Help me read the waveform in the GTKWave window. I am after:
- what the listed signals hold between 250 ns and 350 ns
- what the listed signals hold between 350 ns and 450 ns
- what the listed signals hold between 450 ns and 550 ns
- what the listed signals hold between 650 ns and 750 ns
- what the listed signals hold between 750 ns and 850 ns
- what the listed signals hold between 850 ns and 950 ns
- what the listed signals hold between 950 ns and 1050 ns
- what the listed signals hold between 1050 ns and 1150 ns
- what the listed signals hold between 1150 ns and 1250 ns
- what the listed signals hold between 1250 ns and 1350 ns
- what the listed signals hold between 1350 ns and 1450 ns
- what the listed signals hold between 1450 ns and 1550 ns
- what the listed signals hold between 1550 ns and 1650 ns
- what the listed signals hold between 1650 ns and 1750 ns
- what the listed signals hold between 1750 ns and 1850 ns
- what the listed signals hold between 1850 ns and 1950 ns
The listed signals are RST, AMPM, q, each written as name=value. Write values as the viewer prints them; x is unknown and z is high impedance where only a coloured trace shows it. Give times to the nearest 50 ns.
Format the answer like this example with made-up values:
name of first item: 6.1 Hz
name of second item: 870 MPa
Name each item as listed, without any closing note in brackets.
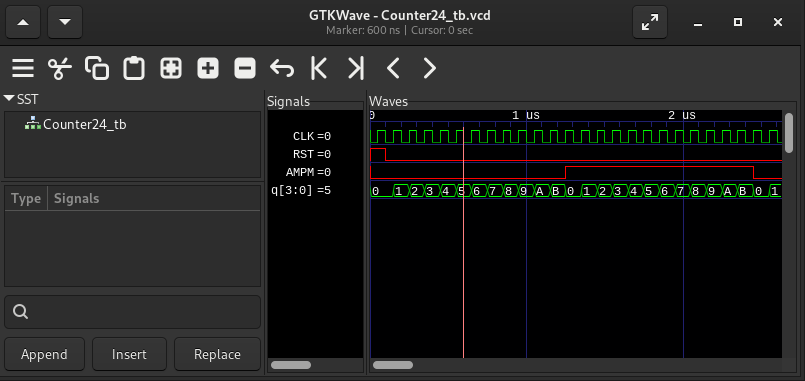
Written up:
what the listed signals hold between 250 ns and 350 ns: RST=0, AMPM=0, q=2
what the listed signals hold between 350 ns and 450 ns: RST=0, AMPM=0, q=3
what the listed signals hold between 450 ns and 550 ns: RST=0, AMPM=0, q=4
what the listed signals hold between 650 ns and 750 ns: RST=0, AMPM=0, q=6
what the listed signals hold between 750 ns and 850 ns: RST=0, AMPM=0, q=7
what the listed signals hold between 850 ns and 950 ns: RST=0, AMPM=0, q=8
what the listed signals hold between 950 ns and 1050 ns: RST=0, AMPM=0, q=9
what the listed signals hold between 1050 ns and 1150 ns: RST=0, AMPM=0, q=A
what the listed signals hold between 1150 ns and 1250 ns: RST=0, AMPM=0, q=B
what the listed signals hold between 1250 ns and 1350 ns: RST=0, AMPM=1, q=0
what the listed signals hold between 1350 ns and 1450 ns: RST=0, AMPM=1, q=1
what the listed signals hold between 1450 ns and 1550 ns: RST=0, AMPM=1, q=2
what the listed signals hold between 1550 ns and 1650 ns: RST=0, AMPM=1, q=3
what the listed signals hold between 1650 ns and 1750 ns: RST=0, AMPM=1, q=4
what the listed signals hold between 1750 ns and 1850 ns: RST=0, AMPM=1, q=5
what the listed signals hold between 1850 ns and 1950 ns: RST=0, AMPM=1, q=6
